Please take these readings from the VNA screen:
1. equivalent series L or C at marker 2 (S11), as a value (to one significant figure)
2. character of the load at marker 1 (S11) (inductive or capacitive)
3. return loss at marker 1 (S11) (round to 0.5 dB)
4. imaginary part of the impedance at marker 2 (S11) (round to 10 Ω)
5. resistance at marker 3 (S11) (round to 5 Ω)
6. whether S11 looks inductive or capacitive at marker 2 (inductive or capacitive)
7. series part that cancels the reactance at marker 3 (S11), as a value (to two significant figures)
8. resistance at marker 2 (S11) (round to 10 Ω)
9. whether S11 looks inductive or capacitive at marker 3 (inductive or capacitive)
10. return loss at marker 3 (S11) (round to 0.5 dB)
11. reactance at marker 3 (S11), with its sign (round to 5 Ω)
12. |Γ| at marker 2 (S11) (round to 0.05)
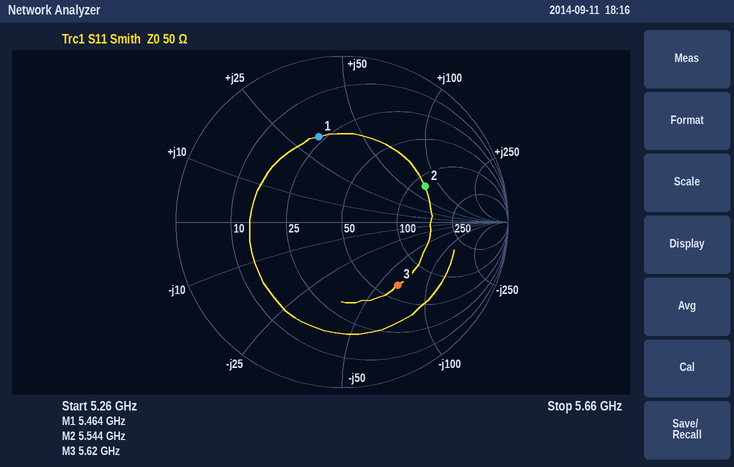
2 nH
inductive
5.5 dB
+70 Ω
65 Ω
inductive
1.8 nH
120 Ω
capacitive
6.0 dB
-65 Ω
0.55
